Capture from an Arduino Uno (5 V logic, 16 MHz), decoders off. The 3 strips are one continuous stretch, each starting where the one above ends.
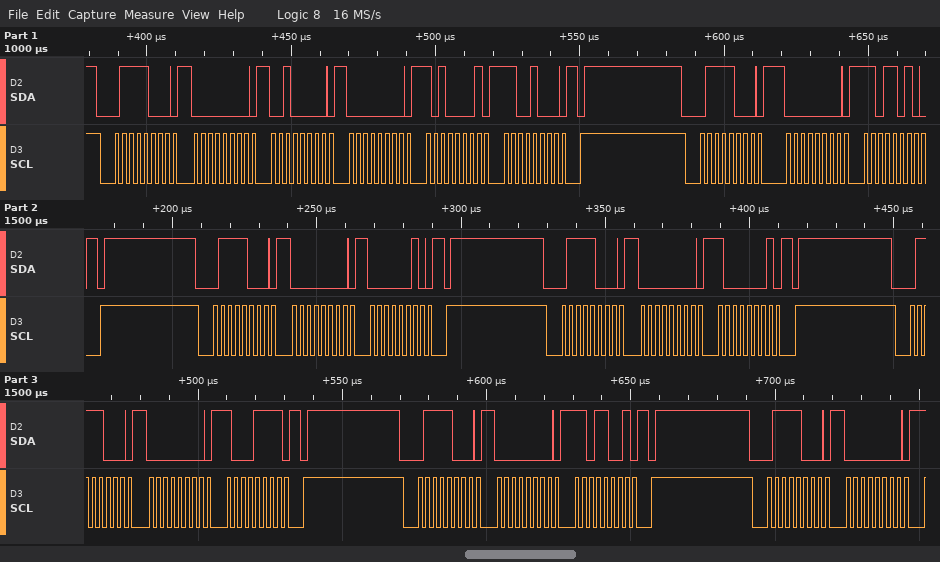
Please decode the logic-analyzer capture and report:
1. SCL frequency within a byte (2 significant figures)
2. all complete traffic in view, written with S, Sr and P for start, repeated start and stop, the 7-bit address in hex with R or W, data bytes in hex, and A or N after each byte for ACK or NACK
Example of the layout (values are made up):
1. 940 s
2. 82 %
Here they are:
1. 400 kHz
2. S 3CW A 00 A 20 A 00 A A1 A C8 A P S 3CW A 00 A DA A P S 3CW A 00 A 02 A P S 3CW A 00 A 81 A P S 3CW A 00 A 8F A P S 3CW A 00 A D9 A P S 3CW A 00 A
